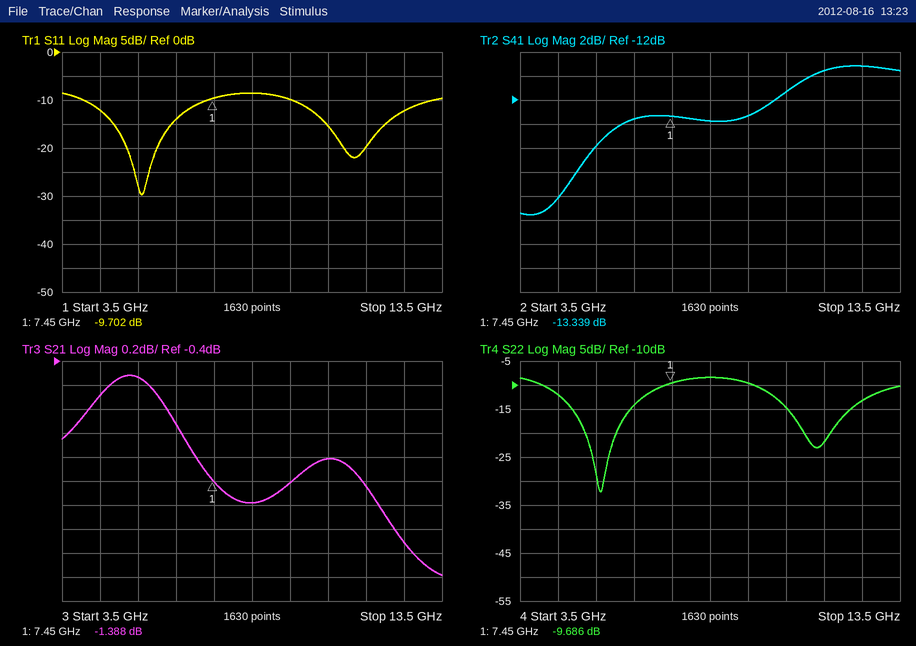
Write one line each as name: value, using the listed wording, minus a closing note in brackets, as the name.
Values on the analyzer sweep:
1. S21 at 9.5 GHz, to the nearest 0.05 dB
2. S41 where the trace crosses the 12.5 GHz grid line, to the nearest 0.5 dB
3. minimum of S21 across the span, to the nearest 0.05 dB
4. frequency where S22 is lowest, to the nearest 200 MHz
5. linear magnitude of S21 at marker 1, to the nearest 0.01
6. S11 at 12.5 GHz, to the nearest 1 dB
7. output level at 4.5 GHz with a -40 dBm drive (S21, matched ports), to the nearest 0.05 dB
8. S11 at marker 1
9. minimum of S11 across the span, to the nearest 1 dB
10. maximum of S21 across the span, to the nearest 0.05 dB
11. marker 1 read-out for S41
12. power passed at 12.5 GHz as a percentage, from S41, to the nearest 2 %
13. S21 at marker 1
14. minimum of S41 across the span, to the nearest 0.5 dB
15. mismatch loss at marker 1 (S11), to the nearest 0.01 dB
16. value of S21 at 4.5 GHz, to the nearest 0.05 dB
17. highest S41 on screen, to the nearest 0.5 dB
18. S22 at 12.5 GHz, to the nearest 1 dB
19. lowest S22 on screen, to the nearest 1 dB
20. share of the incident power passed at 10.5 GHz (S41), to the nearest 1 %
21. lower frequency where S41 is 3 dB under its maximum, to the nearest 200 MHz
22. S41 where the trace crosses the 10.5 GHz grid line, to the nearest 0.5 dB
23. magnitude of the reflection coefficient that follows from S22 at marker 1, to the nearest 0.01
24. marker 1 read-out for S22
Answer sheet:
S21 at 9.5 GHz, to the nearest 0.05 dB: -1.40 dB
S41 where the trace crosses the 12.5 GHz grid line, to the nearest 0.5 dB: -9.0 dB
minimum of S21 across the span, to the nearest 0.05 dB: -2.20 dB
frequency where S22 is lowest, to the nearest 200 MHz: 5.6 GHz
linear magnitude of S21 at marker 1, to the nearest 0.01: 0.85
S11 at 12.5 GHz, to the nearest 1 dB: -12 dB
output level at 4.5 GHz with a -40 dBm drive (S21, matched ports), to the nearest 0.05 dB: -40.70 dBm
S11 at marker 1: -9.702 dB
minimum of S11 across the span, to the nearest 1 dB: -30 dB
maximum of S21 across the span, to the nearest 0.05 dB: -0.50 dB
marker 1 read-out for S41: -13.339 dB
power passed at 12.5 GHz as a percentage, from S41, to the nearest 2 %: 12 %
S21 at marker 1: -1.388 dB
minimum of S41 across the span, to the nearest 0.5 dB: -21.5 dB
mismatch loss at marker 1 (S11), to the nearest 0.01 dB: 0.49 dB
value of S21 at 4.5 GHz, to the nearest 0.05 dB: -0.70 dB
highest S41 on screen, to the nearest 0.5 dB: -9.0 dB
S22 at 12.5 GHz, to the nearest 1 dB: -13 dB
lowest S22 on screen, to the nearest 1 dB: -32 dB
share of the incident power passed at 10.5 GHz (S41), to the nearest 1 %: 7 %
lower frequency where S41 is 3 dB under its maximum, to the nearest 200 MHz: 10.2 GHz
S41 where the trace crosses the 10.5 GHz grid line, to the nearest 0.5 dB: -11.5 dB
magnitude of the reflection coefficient that follows from S22 at marker 1, to the nearest 0.01: 0.33
marker 1 read-out for S22: -9.686 dB
